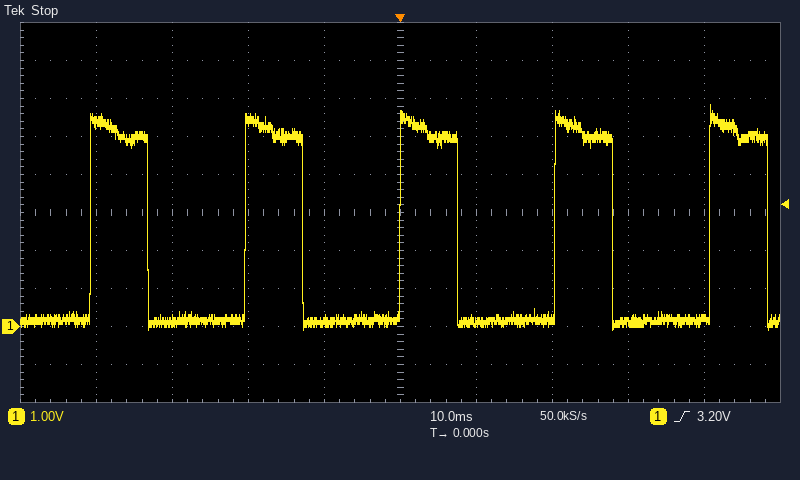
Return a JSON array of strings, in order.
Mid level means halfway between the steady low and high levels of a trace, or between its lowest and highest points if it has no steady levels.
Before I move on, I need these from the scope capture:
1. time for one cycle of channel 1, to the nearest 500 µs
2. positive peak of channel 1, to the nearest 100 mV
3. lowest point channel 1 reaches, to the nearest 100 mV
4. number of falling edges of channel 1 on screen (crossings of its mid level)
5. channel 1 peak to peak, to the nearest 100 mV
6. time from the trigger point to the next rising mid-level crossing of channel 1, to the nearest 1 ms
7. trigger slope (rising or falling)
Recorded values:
["20.5 ms", "5.8 V", "-100 mV", "5", "5.9 V", "20 ms", "rising"]
